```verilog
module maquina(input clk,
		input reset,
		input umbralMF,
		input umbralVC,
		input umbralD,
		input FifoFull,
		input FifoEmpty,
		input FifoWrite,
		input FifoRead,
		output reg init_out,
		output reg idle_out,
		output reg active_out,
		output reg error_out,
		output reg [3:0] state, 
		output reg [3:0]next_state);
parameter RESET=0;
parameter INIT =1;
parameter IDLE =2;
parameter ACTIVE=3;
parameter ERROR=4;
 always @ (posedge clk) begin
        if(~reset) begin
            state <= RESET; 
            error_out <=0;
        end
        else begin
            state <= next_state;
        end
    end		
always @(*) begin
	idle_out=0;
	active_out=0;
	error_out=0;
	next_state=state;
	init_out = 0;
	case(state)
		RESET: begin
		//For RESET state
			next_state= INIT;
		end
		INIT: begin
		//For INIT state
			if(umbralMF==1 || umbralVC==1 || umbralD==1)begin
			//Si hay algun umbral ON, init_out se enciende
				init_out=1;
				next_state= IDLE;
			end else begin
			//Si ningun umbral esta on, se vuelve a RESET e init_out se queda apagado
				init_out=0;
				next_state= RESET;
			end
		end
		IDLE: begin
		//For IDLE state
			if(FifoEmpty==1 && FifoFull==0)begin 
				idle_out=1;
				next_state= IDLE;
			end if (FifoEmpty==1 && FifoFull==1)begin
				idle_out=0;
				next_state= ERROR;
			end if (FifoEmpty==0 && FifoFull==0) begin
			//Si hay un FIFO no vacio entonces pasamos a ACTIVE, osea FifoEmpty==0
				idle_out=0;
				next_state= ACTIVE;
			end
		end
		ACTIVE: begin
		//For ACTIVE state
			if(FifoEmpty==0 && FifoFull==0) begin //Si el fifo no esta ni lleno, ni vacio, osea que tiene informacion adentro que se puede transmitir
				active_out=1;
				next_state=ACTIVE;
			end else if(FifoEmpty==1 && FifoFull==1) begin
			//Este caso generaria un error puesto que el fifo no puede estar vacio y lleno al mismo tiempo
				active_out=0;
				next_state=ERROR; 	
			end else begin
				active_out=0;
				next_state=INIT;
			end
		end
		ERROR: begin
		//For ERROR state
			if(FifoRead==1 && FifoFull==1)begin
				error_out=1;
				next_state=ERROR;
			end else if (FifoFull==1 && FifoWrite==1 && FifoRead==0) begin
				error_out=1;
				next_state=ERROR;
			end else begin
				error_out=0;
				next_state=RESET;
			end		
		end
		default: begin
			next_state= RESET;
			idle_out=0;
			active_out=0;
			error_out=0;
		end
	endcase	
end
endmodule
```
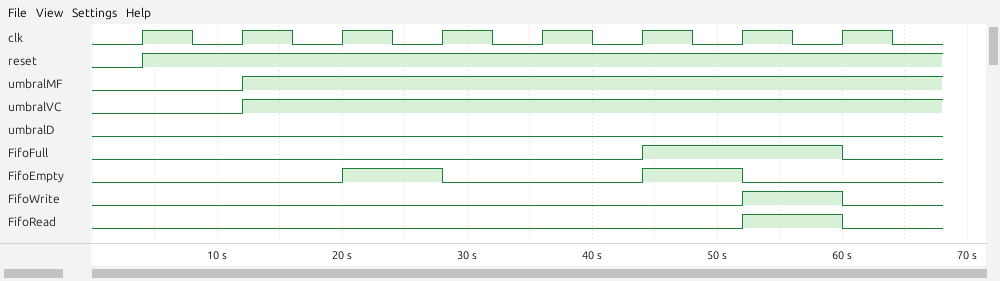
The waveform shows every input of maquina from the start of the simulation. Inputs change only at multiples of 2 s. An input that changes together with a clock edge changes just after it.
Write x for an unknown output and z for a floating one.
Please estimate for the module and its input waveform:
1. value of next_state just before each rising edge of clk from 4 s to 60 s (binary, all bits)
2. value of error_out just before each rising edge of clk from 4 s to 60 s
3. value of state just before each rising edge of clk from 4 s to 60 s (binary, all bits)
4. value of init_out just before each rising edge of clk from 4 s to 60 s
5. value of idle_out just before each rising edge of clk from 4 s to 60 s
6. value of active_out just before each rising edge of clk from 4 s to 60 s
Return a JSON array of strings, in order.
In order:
["0000, 0001, 0010, 0010, 0011, 0011, 0100, 0100", "0 0 0 0 0 0 0 1", "x, 0000, 0001, 0010, 0010, 0011, 0011, 0100", "0 0 1 0 0 0 0 0", "0 0 0 1 0 0 0 0", "0 0 0 0 0 1 0 0"]
